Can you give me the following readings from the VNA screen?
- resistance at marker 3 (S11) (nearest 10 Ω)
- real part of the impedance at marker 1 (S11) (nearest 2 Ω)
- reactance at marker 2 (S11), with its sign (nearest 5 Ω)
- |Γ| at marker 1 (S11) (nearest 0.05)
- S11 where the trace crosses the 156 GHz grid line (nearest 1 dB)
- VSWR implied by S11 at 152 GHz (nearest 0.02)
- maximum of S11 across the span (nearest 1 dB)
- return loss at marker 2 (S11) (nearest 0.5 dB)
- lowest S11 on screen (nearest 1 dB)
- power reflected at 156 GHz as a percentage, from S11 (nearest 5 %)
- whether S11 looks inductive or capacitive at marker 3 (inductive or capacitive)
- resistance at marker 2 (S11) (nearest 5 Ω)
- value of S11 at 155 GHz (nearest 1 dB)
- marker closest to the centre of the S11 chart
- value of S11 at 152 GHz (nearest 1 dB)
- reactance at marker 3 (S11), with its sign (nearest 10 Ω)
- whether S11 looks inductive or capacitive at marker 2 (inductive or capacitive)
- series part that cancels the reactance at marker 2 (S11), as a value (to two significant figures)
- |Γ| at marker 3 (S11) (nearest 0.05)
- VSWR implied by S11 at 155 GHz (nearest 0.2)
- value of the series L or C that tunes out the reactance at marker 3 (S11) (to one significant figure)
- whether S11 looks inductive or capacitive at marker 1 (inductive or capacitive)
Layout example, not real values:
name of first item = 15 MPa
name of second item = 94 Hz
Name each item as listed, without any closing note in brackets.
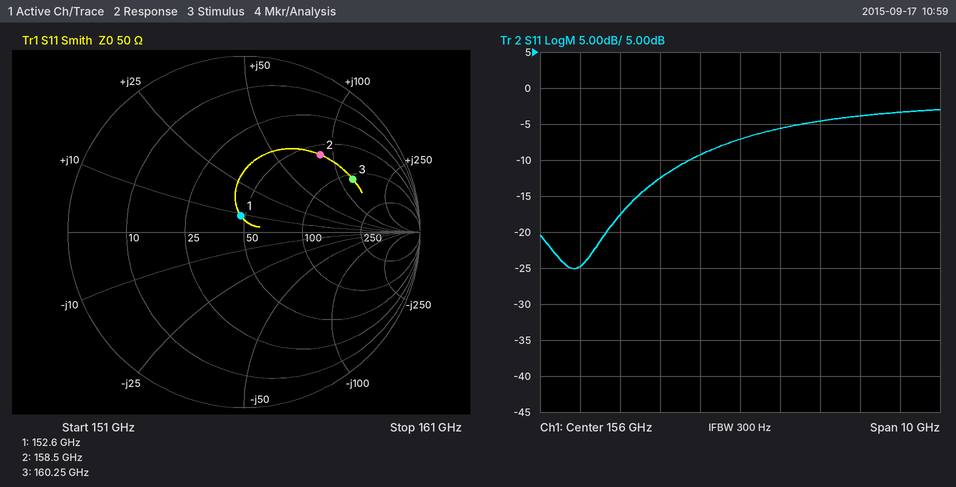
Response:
resistance at marker 3 (S11) = 110 Ω
real part of the impedance at marker 1 (S11) = 48 Ω
reactance at marker 2 (S11), with its sign = +85 Ω
|Γ| at marker 1 (S11) = 0.10
S11 where the trace crosses the 156 GHz grid line = -7 dB
VSWR implied by S11 at 152 GHz = 1.12
maximum of S11 across the span = -3 dB
return loss at marker 2 (S11) = 4.0 dB
lowest S11 on screen = -25 dB
power reflected at 156 GHz as a percentage, from S11 = 20 %
whether S11 looks inductive or capacitive at marker 3 = inductive
resistance at marker 2 (S11) = 60 Ω
value of S11 at 155 GHz = -9 dB
marker closest to the centre of the S11 chart = marker 1
value of S11 at 152 GHz = -25 dB
reactance at marker 3 (S11), with its sign = +130 Ω
whether S11 looks inductive or capacitive at marker 2 = inductive
series part that cancels the reactance at marker 2 (S11), as a value = 12 fF
|Γ| at marker 3 (S11) = 0.70
VSWR implied by S11 at 155 GHz = 2.0
value of the series L or C that tunes out the reactance at marker 3 (S11) = 8 fF
whether S11 looks inductive or capacitive at marker 1 = inductive
